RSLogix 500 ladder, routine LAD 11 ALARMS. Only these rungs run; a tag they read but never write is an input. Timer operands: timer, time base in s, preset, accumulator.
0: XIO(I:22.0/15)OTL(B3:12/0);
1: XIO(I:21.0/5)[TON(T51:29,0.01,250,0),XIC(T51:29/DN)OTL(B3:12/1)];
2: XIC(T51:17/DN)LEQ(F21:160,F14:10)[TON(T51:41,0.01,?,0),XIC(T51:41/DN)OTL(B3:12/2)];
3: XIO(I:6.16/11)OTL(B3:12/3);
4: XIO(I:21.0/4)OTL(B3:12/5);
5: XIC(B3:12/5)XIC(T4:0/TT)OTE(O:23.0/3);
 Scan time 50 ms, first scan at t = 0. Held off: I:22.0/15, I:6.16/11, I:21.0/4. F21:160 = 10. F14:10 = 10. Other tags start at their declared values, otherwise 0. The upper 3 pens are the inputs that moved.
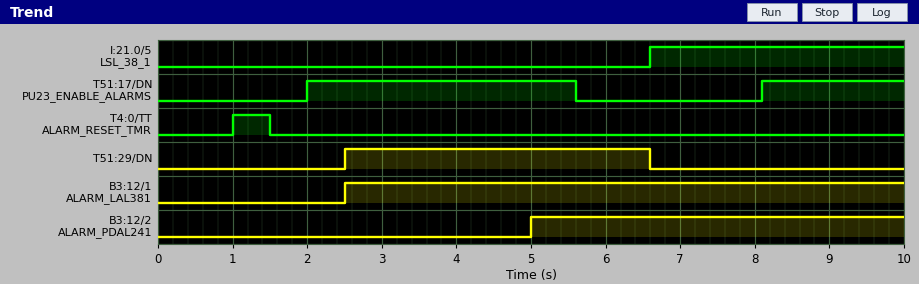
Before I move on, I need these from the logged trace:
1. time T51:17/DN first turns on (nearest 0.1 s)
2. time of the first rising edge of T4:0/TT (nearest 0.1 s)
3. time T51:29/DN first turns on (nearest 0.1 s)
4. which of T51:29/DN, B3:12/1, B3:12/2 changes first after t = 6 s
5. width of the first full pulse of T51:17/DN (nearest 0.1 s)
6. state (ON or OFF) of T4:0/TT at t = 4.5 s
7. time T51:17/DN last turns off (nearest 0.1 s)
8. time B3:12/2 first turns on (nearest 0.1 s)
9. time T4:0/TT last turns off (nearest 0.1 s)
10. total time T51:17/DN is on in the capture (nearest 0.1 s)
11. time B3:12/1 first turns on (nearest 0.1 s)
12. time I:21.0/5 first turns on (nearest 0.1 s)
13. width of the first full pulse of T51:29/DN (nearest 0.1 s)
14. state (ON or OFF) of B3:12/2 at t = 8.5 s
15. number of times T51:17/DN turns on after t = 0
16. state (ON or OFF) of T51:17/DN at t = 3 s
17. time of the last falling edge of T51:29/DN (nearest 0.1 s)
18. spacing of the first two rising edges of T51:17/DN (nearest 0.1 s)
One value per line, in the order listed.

2.0 s
1.0 s
2.5 s
T51:29/DN
3.6 s
OFF
5.6 s
5.0 s
1.5 s
5.5 s
2.5 s
6.6 s
4.1 s
ON
2
ON
6.6 s
6.1 s
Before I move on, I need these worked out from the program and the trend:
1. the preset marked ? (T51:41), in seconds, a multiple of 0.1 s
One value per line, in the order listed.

3.0 s
